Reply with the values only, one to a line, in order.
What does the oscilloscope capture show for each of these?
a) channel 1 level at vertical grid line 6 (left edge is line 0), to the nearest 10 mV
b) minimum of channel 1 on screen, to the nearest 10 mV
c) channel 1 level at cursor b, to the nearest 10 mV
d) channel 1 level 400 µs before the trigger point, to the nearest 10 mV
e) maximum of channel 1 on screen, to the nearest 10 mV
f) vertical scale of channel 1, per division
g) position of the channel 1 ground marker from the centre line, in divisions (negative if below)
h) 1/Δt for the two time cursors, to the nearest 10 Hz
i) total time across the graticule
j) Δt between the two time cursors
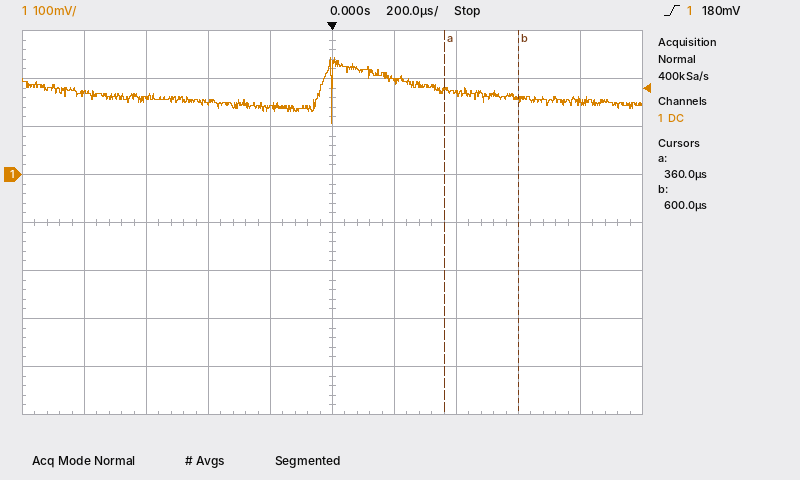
200 mV
110 mV
160 mV
150 mV
240 mV
100 mV
+1.0 div
4.17 kHz
2 ms
240 µs
